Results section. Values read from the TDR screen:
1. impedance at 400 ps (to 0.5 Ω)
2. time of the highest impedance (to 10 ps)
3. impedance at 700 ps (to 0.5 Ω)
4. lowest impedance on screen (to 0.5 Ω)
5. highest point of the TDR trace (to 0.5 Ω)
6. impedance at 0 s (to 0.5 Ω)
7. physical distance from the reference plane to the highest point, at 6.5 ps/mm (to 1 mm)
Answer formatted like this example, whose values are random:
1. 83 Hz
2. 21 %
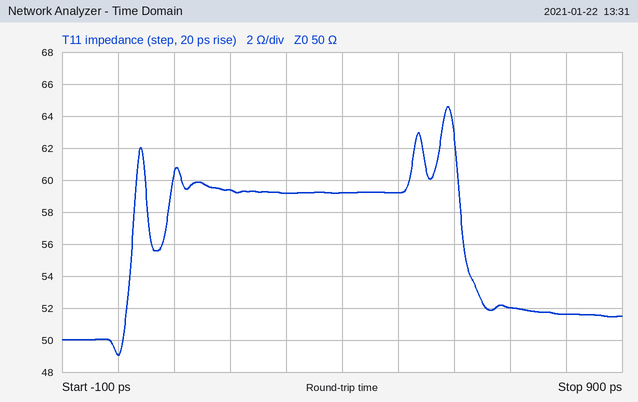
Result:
1. 59.0 Ω
2. 590 ps
3. 52.0 Ω
4. 49.0 Ω
5. 64.5 Ω
6. 49.0 Ω
7. 45 mm
